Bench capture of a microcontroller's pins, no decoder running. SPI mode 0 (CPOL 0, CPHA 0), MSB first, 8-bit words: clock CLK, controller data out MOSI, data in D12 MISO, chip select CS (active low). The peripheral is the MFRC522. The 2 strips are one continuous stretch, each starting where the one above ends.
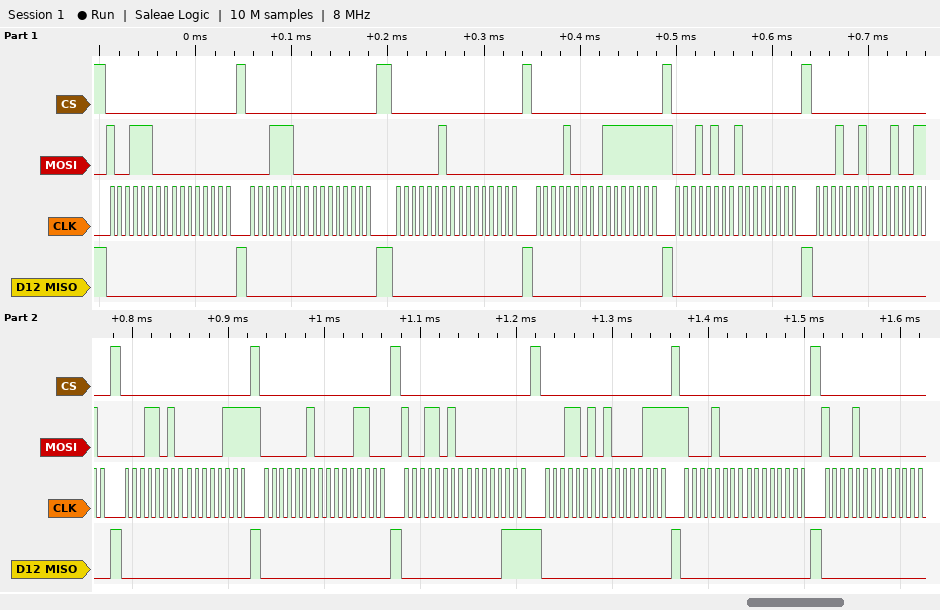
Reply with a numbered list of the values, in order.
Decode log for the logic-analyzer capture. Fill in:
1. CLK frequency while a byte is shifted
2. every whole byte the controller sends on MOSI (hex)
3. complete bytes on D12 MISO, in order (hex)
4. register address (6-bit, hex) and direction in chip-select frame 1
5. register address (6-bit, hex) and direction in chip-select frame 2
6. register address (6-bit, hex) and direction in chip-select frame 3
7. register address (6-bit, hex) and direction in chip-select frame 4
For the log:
1. 125 kHz
2. 0x9C 0x00 0x1C 0x00 0x02 0x00 0x08 0x7F 0x14 0x80 0x12 0x26 0x1A 0x07 0x02 0x0C 0x9A 0x00 0x1A 0x87 0x88 0x00 0x88
3. 0x00 0x00 0x00 0x00 0x00 0x00 0x00 0x00 0x00 0x00 0x00 0x00 0x00 0x00 0x00 0x00 0x00 0x07 0x00 0x00 0x00 0x00 0x00
4. 0x0E read
5. 0x0E write
6. 0x01 write
7. 0x04 write
